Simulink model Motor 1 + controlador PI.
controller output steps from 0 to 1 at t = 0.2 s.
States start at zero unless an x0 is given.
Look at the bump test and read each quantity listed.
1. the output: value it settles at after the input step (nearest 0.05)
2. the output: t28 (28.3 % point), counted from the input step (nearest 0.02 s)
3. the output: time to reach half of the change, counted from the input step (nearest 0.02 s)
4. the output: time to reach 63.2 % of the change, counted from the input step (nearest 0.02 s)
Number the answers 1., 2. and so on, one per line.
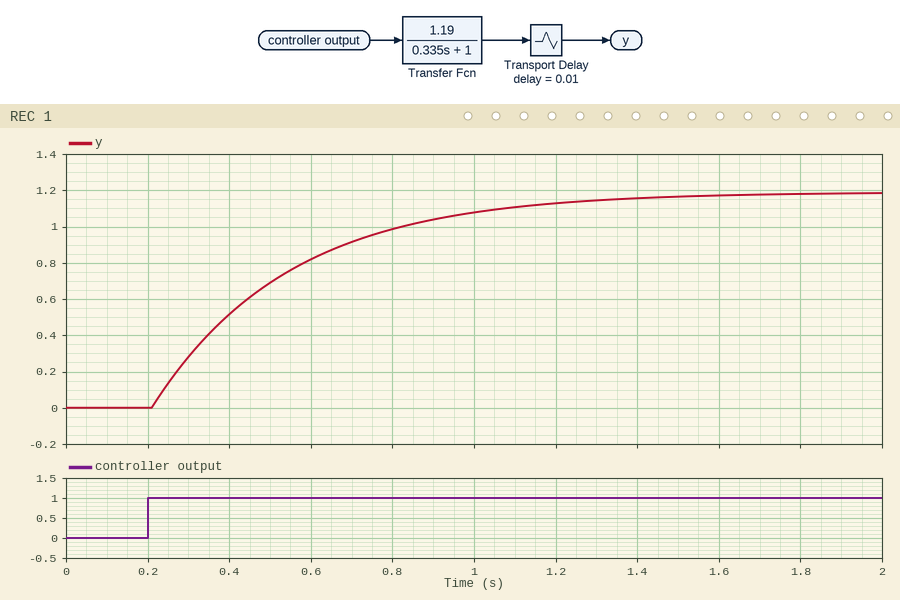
1. 1.20
2. 0.12 s
3. 0.24 s
4. 0.34 s
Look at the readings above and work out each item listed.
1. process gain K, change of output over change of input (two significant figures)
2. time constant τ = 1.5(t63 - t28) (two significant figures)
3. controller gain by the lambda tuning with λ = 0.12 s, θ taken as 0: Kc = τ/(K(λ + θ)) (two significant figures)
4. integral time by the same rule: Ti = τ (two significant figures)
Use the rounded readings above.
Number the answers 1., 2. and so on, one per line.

1. 1.2
2. 0.33 s
3. 2.3
4. 0.33 s
